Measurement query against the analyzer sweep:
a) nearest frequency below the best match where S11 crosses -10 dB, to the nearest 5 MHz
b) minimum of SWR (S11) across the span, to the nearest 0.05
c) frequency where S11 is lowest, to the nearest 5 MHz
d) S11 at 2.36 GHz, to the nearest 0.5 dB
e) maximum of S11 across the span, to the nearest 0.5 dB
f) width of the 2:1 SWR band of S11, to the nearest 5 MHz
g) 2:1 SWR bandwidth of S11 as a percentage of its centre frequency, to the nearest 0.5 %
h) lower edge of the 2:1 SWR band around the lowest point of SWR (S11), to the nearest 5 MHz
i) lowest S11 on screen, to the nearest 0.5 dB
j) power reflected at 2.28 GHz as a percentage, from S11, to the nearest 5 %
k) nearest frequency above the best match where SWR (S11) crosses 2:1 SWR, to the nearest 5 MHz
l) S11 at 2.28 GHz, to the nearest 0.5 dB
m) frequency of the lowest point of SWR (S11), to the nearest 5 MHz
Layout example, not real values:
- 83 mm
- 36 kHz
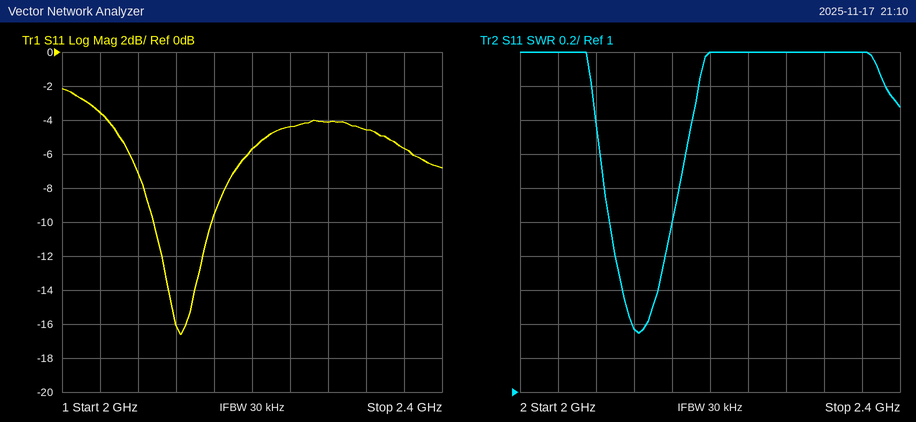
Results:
- 2.095 GHz
- 1.35
- 2.125 GHz
- -5.5 dB
- -2.0 dB
- 65 MHz
- 3.0 %
- 2.095 GHz
- -16.5 dB
- 40 %
- 2.160 GHz
- -4.0 dB
- 2.125 GHz
